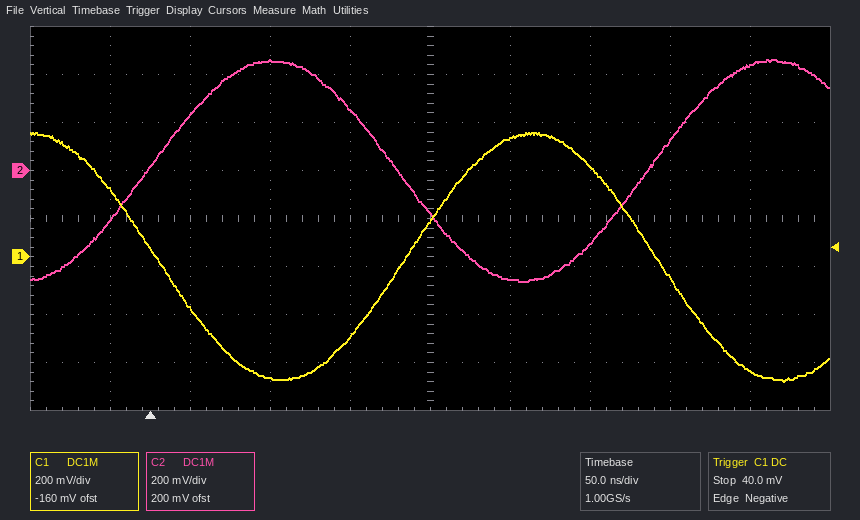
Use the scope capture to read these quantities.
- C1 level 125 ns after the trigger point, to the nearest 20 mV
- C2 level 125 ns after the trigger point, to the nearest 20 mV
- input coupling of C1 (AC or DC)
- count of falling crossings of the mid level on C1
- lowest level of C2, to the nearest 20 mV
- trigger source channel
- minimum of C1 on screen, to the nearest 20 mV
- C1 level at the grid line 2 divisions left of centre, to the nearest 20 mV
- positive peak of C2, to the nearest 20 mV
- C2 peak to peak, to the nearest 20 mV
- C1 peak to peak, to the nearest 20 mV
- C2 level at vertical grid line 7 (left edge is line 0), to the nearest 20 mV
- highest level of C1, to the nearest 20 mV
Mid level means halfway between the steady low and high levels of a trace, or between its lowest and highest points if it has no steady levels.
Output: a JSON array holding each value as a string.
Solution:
["-340 mV", "260 mV", "DC", "2", "-460 mV", "C1", "-520 mV", "-500 mV", "460 mV", "920 mV", "1.04 V", "-300 mV", "520 mV"]
